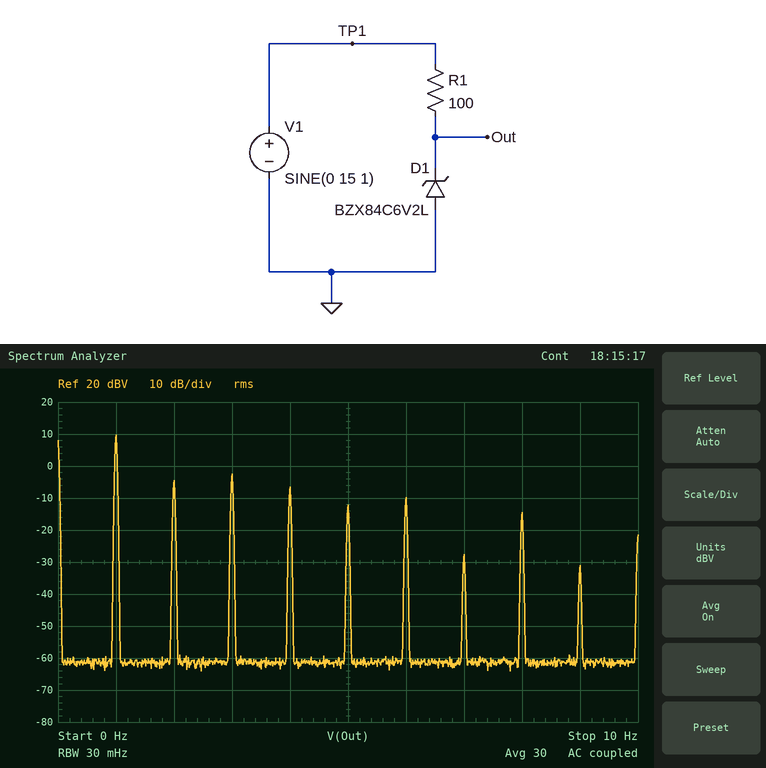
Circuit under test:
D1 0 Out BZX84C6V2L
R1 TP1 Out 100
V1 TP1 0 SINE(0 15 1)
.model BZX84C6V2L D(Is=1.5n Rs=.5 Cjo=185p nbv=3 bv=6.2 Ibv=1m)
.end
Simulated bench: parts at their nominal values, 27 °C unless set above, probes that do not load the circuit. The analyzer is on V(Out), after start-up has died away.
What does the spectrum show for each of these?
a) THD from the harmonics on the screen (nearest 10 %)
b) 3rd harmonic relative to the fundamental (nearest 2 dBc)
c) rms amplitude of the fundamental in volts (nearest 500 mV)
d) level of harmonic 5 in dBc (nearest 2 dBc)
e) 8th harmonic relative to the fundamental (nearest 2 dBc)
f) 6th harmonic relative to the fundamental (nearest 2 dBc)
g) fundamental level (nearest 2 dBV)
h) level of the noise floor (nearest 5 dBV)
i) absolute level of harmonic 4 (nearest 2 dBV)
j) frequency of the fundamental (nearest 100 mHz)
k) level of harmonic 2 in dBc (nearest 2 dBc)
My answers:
40 %
-12 dBc
3.0 V
-22 dBc
-24 dBc
-20 dBc
10 dBV
-60 dBV
-6 dBV
1.0 Hz
-14 dBc
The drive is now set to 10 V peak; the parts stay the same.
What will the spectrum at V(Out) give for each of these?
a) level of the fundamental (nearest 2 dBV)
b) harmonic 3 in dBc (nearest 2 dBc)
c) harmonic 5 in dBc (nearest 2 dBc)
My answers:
10 dBV
-16 dBc
-44 dBc
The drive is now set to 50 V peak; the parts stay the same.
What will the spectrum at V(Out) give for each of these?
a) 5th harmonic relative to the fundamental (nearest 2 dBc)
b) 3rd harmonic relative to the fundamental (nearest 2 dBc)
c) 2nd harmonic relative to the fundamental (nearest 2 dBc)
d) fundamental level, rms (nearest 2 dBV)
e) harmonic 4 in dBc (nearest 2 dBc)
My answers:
-16 dBc
-10 dBc
-24 dBc
10 dBV
-24 dBc
